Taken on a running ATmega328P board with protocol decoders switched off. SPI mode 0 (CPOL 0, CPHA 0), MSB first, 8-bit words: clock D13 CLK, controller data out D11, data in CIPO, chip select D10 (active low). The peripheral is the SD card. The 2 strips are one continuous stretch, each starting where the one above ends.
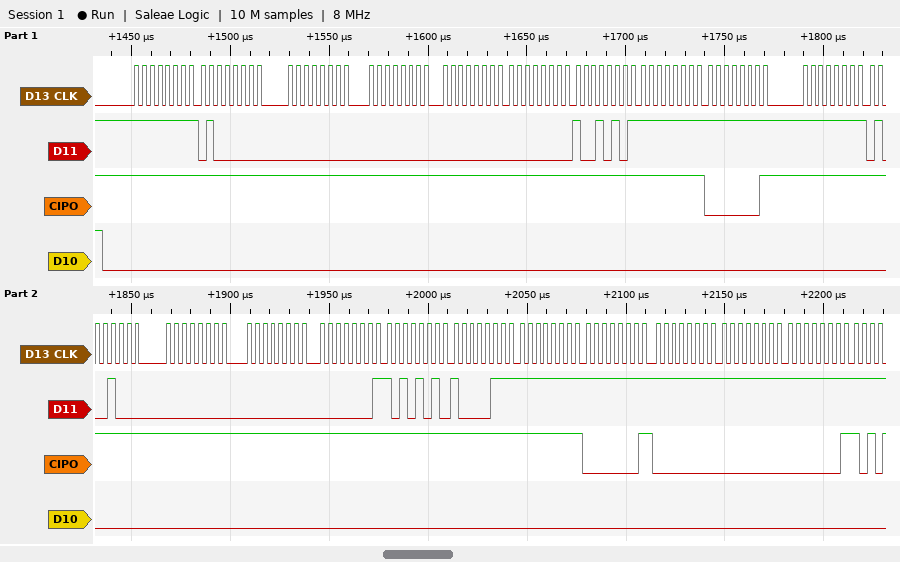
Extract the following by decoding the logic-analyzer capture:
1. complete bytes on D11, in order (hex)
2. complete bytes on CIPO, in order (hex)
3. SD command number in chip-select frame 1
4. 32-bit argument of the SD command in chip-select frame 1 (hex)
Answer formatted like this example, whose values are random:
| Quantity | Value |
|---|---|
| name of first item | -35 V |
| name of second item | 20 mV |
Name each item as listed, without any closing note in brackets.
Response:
| Quantity | Value |
|---|---|
| complete bytes on D11, in order | 0xFF 0x40 0x00 0x00 0x00 0x00 0x95 0xFF 0xFF 0xFF 0x48 0x00 0x00 0x01 0xAA 0x87 0xFF 0xFF 0xFF 0xFF 0xFF |
| complete bytes on CIPO, in order | 0xFF 0xFF 0xFF 0xFF 0xFF 0xFF 0xFF 0xFF 0x01 0xFF 0xFF 0xFF 0xFF 0xFF 0xFF 0xFF 0xFF 0x01 0x00 0x00 0x01 |
| SD command number in chip-select frame 1 | CMD0 |
| 32-bit argument of the SD command in chip-select frame 1 | 0x00000000 |
